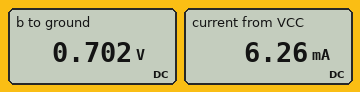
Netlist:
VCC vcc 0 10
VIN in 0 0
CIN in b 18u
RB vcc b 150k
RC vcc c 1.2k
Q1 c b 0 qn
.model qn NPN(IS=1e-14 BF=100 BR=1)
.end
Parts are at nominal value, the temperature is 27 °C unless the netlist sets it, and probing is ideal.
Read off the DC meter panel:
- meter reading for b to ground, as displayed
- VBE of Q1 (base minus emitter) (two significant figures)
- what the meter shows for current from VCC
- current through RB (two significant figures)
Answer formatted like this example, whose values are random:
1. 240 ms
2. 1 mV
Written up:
1. 0.702 V
2. 700 mV
3. 6.26 mA
4. 62 µA
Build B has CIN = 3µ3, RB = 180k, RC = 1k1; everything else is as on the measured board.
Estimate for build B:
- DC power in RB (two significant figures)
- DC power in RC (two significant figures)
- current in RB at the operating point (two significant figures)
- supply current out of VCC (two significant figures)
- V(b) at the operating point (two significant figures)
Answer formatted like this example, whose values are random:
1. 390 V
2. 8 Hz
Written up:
1. 480 µW
2. 29 mW
3. 52 µA
4. 5.2 mA
5. 700 mV
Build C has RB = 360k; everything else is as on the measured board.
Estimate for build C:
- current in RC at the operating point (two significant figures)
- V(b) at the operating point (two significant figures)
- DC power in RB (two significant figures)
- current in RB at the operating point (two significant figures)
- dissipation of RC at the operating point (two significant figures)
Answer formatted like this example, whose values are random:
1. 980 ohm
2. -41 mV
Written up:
1. 2.6 mA
2. 680 mV
3. 240 µW
4. 26 µA
5. 8.0 mW
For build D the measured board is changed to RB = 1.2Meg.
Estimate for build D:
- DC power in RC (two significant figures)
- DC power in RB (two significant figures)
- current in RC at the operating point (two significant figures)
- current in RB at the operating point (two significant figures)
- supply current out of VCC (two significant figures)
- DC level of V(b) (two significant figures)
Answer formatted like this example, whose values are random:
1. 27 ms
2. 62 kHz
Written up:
1. 730 µW
2. 73 µW
3. 780 µA
4. 7.8 µA
5. 790 µA
6. 650 mV
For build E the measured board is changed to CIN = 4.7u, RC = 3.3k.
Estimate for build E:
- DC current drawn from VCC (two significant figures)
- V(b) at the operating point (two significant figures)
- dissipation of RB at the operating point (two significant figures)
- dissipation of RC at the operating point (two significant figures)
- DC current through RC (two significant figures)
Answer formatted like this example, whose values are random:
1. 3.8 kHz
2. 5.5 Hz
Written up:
1. 3.1 mA
2. 680 mV
3. 580 µW
4. 30 mW
5. 3.0 mA
